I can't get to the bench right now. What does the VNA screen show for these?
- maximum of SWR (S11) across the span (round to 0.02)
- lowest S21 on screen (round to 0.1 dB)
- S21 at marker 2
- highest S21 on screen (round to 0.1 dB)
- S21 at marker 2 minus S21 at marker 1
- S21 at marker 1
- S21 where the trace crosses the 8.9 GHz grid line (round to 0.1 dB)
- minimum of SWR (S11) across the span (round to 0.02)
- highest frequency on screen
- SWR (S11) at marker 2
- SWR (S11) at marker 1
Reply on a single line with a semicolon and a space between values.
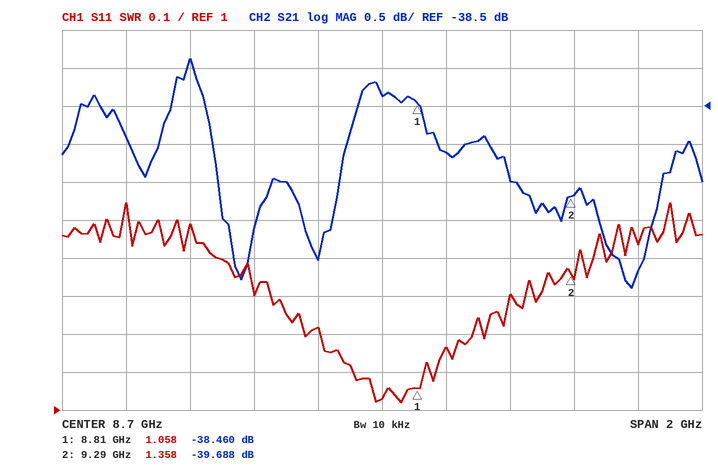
1.54; -40.9 dB; -39.688 dB; -37.9 dB; -1.228 dB; -38.460 dB; -39.1 dB; 1.02; 9.7 GHz; 1.358; 1.058
